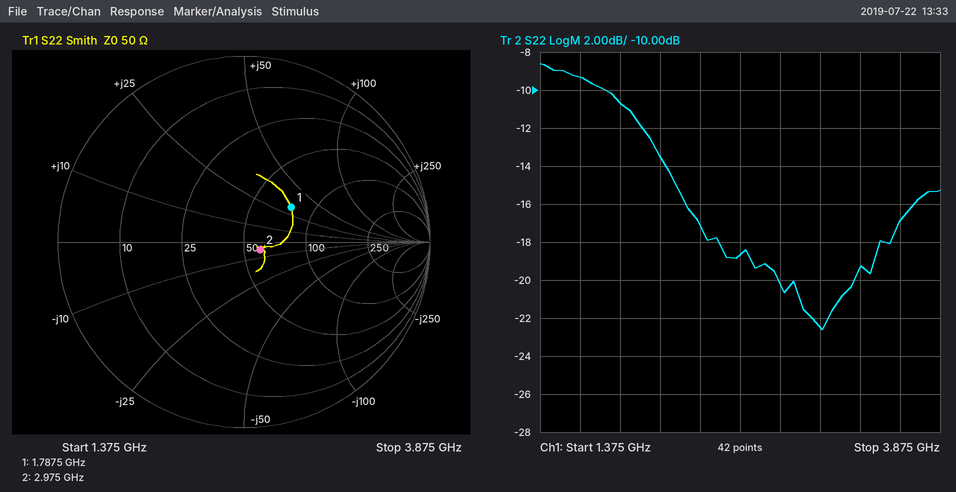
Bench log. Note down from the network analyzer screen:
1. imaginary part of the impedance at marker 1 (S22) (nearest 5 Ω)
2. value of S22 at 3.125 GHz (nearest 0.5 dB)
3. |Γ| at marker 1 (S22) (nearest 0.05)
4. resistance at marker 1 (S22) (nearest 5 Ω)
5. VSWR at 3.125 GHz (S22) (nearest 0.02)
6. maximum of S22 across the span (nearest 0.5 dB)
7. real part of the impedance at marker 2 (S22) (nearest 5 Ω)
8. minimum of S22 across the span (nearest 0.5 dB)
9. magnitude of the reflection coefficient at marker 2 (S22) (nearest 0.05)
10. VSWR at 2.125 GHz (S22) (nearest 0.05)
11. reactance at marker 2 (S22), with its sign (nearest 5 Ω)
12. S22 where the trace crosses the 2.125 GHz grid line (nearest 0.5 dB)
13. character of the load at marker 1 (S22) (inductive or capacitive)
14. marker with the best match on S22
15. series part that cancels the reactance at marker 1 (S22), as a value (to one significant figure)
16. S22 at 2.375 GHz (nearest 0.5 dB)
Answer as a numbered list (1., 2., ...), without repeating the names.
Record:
1. +30 Ω
2. -22.5 dB
3. 0.30
4. 75 Ω
5. 1.16
6. -8.5 dB
7. 60 Ω
8. -22.5 dB
9. 0.10
10. 1.55
11. -5 Ω
12. -13.5 dB
13. inductive
14. marker 2
15. 3 pF
16. -17.0 dB
